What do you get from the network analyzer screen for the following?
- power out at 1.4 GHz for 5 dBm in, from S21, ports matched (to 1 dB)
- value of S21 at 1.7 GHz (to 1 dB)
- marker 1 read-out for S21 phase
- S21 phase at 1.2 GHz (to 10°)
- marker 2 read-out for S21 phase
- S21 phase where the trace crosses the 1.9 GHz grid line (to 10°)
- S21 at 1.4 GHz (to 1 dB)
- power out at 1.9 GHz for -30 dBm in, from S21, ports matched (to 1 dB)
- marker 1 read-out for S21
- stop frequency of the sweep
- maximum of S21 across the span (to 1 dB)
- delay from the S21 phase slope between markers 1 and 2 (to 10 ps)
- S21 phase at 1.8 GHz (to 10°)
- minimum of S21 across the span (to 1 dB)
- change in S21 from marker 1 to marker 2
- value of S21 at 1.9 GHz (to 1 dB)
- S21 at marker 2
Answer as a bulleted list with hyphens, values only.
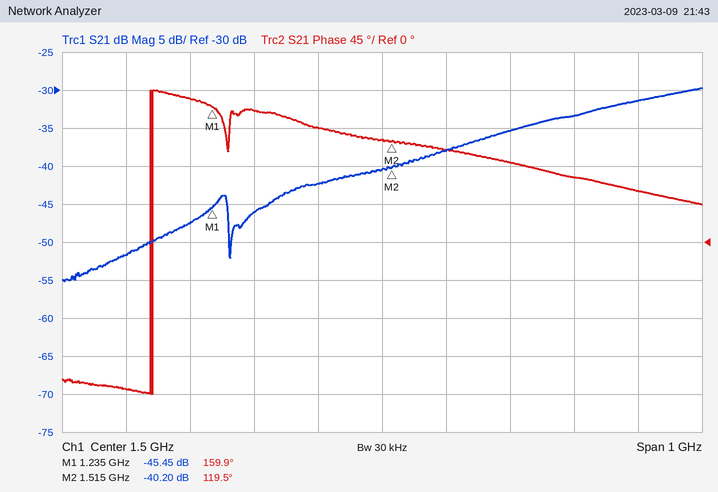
- -37 dBm
- -35 dB
- 159.9°
- 170°
- 119.5°
- 60°
- -42 dB
- -61 dBm
- -45.45 dB
- 2 GHz
- -30 dB
- 400 ps
- 80°
- -55 dB
- 5.25 dB
- -31 dB
- -40.20 dB
